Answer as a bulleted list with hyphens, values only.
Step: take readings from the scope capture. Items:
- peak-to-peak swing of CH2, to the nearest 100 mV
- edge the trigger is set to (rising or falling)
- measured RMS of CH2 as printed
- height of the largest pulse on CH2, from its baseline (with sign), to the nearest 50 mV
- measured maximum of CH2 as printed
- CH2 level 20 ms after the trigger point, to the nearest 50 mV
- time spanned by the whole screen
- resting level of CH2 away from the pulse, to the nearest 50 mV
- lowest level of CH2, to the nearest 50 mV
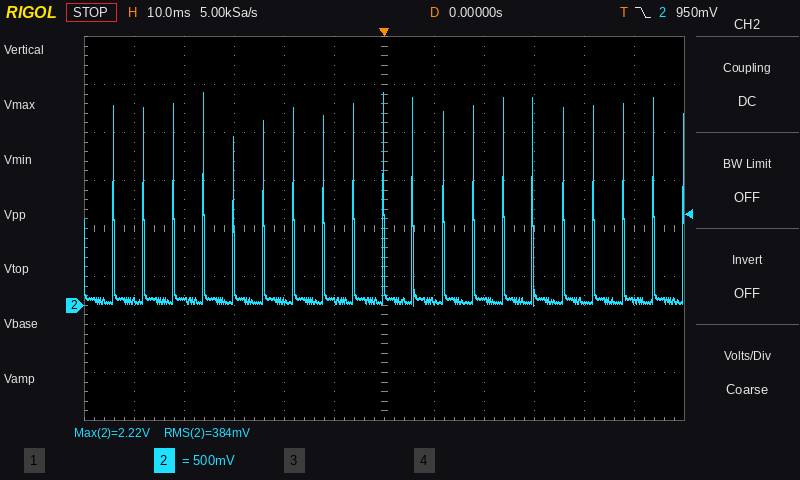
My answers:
- 2.20 V
- falling
- 384 mV
- +2.15 V
- 2.22 V
- 50 mV
- 120 ms
- 50 mV
- 0 mV
